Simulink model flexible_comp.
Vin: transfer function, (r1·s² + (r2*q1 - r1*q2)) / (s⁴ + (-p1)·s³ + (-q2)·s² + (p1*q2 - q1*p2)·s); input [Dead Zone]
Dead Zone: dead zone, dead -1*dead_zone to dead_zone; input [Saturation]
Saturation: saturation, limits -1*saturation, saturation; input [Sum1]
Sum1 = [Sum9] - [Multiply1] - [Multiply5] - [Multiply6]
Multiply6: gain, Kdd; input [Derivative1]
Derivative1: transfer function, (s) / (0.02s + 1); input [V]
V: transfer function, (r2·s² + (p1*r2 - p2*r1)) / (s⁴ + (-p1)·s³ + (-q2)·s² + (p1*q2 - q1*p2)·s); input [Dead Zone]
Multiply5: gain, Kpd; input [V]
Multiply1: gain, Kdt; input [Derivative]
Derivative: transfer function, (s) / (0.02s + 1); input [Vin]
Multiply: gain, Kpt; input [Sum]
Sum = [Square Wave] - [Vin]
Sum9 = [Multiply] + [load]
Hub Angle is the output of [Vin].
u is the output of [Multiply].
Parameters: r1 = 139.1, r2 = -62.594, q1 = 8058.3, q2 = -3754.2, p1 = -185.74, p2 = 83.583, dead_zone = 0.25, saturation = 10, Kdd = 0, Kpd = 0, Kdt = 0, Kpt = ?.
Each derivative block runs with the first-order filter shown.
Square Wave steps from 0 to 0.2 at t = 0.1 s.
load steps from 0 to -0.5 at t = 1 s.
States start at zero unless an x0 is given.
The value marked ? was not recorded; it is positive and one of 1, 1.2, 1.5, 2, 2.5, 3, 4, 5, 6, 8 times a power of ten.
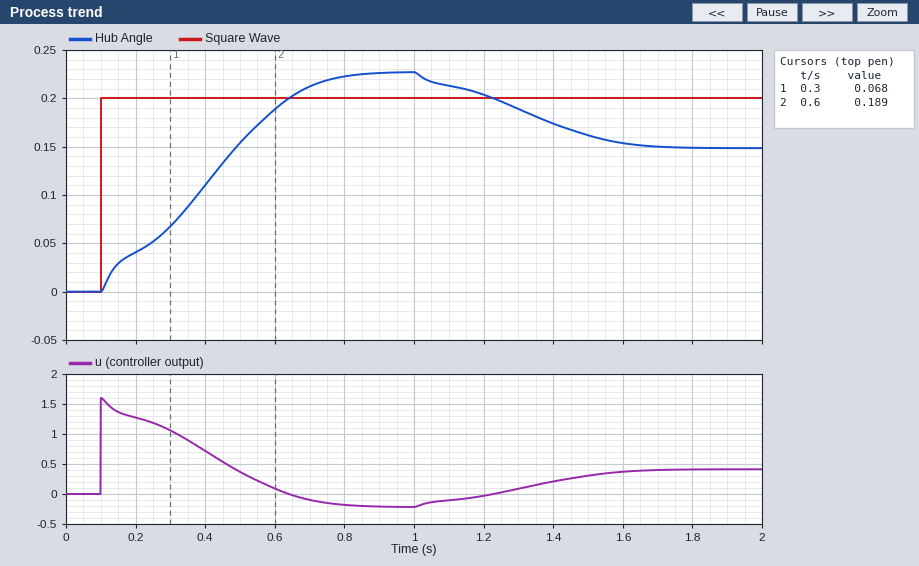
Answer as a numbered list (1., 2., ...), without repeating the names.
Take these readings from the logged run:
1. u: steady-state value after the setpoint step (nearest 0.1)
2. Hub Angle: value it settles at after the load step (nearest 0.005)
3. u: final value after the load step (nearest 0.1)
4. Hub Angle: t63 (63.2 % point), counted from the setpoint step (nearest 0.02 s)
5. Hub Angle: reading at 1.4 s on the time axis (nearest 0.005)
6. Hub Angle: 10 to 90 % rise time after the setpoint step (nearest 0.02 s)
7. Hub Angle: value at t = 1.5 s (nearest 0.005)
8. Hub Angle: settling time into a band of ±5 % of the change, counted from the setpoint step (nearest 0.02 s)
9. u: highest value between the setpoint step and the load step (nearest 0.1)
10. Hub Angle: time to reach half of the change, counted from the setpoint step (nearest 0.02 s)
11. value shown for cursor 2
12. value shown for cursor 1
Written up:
1. -0.2
2. 0.150
3. 0.4
4. 0.38 s
5. 0.175
6. 0.52 s
7. 0.160
8. 0.62 s
9. 1.6
10. 0.30 s
11. 0.189
12. 0.068
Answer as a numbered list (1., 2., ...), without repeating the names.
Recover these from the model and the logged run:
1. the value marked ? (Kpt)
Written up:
1. 8
